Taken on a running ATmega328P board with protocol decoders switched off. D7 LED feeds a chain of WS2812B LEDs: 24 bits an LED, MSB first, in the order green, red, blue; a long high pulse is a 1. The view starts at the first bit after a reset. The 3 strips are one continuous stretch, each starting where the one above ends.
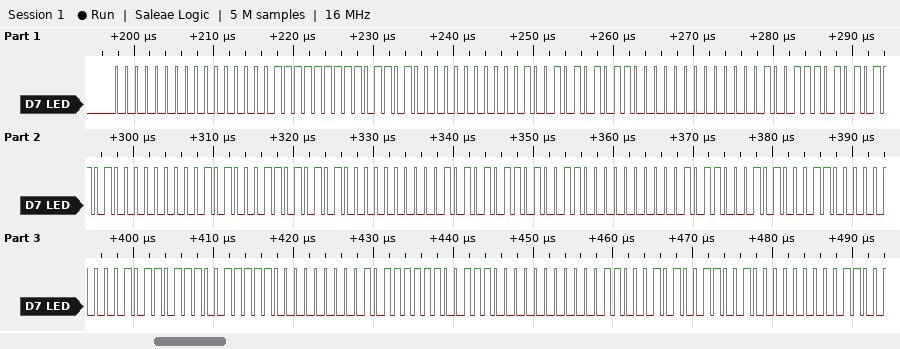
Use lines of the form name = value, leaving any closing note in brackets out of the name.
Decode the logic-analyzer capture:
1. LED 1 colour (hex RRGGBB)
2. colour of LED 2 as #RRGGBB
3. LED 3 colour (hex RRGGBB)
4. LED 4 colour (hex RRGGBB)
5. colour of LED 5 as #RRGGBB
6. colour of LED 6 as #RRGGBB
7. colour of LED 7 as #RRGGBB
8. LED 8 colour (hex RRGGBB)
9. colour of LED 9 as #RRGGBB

LED 1 colour = #0000FF
colour of LED 2 as #RRGGBB = #00B44A
LED 3 colour = #00B04E
LED 4 colour = #00AD51
colour of LED 5 as #RRGGBB = #00AA55
colour of LED 6 as #RRGGBB = #00A658
colour of LED 7 as #RRGGBB = #00A35B
LED 8 colour = #009F5F
colour of LED 9 as #RRGGBB = #009C62
